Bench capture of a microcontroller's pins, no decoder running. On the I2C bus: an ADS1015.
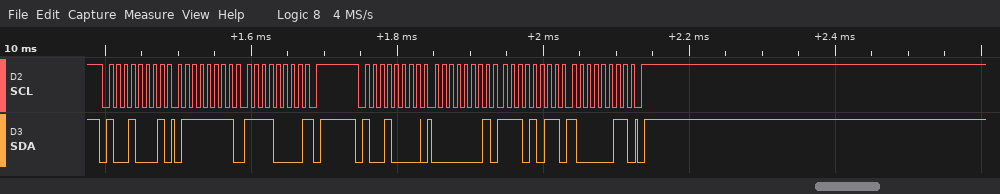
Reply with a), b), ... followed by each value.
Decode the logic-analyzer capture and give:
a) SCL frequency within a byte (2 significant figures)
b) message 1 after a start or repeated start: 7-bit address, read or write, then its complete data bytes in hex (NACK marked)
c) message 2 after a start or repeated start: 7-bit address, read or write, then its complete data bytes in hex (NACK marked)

a) 100 kHz
b) 0x48 read: 7F F0 NACK
c) 0x48 write: 01 EB 83
